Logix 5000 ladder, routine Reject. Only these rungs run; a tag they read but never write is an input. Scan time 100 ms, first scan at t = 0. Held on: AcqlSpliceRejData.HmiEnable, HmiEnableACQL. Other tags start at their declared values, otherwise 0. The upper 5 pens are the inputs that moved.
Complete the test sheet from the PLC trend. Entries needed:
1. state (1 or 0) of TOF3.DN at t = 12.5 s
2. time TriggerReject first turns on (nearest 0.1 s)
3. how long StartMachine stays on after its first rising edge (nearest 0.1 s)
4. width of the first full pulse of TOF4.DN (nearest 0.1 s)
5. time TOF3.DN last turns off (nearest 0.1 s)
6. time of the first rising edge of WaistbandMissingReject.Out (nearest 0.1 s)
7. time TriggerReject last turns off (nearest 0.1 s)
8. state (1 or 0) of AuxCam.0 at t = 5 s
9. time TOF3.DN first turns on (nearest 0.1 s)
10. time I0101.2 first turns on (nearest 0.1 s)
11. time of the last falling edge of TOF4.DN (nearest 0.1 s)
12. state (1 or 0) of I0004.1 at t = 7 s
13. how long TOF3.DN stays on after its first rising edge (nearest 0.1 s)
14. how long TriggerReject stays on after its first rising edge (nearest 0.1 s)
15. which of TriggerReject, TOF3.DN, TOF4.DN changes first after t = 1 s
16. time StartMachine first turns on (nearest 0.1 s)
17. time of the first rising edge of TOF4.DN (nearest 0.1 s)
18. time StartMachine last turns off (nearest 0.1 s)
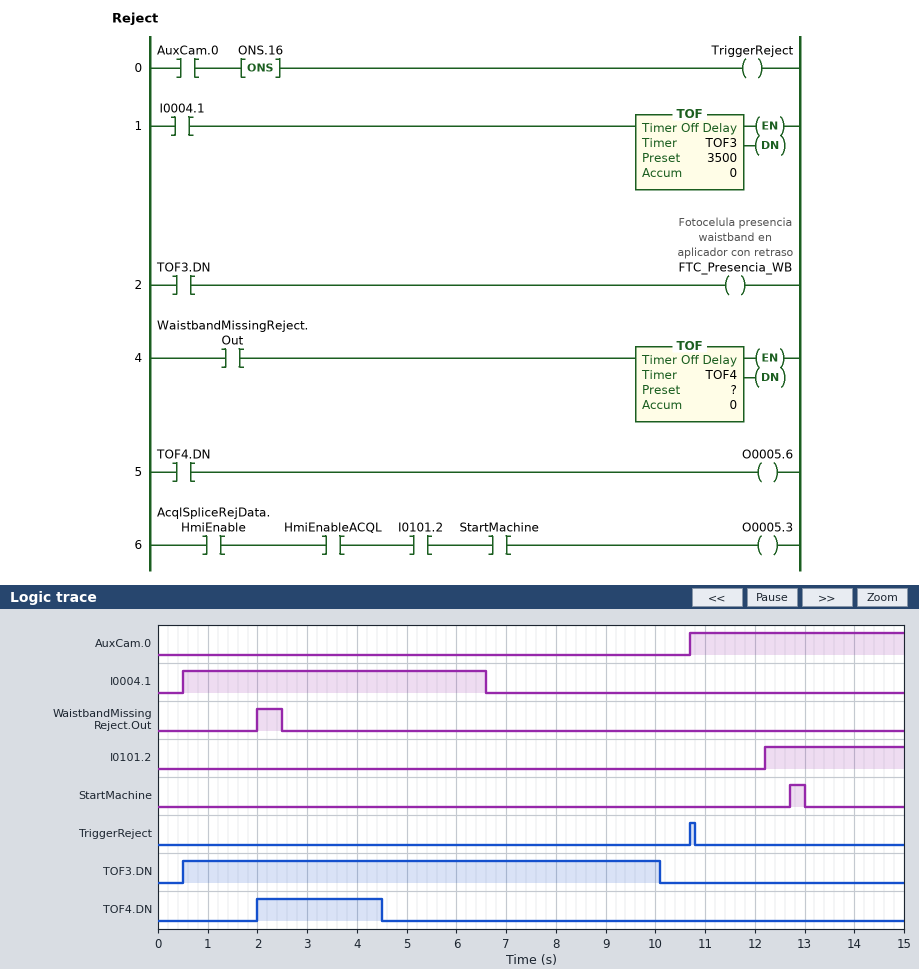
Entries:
0
10.7 s
0.3 s
2.5 s
10.1 s
2.0 s
10.8 s
0
0.5 s
12.2 s
4.5 s
0
9.6 s
0.1 s
TOF4.DN
12.7 s
2.0 s
13.0 s
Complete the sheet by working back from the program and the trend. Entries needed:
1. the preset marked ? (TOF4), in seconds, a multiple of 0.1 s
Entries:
2.0 s
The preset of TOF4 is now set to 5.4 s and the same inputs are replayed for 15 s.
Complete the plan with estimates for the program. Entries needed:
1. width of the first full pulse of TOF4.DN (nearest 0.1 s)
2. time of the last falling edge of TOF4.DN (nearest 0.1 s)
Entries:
5.9 s
7.9 s
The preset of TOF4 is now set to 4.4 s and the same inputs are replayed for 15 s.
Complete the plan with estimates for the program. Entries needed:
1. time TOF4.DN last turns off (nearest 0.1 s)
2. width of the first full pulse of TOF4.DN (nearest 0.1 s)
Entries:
6.9 s
4.9 s
